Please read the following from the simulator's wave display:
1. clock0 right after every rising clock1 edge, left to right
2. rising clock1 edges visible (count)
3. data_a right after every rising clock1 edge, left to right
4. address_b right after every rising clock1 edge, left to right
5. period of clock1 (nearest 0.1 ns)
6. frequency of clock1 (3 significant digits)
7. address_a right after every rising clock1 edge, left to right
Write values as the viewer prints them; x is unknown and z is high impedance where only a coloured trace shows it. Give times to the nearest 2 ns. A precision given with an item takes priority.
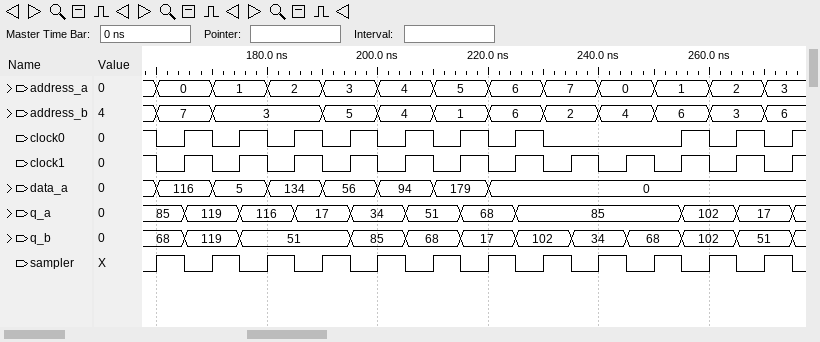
1 1 1 1 1 1 1 0 0 1 1 1
12
116, 5, 134, 56, 94, 179, 0, 0, 0, 0, 0, 0
7, 3, 3, 5, 4, 1, 6, 2, 4, 6, 3, 6
10 ns
100 MHz
0, 1, 2, 3, 4, 5, 6, 7, 0, 1, 2, 3
